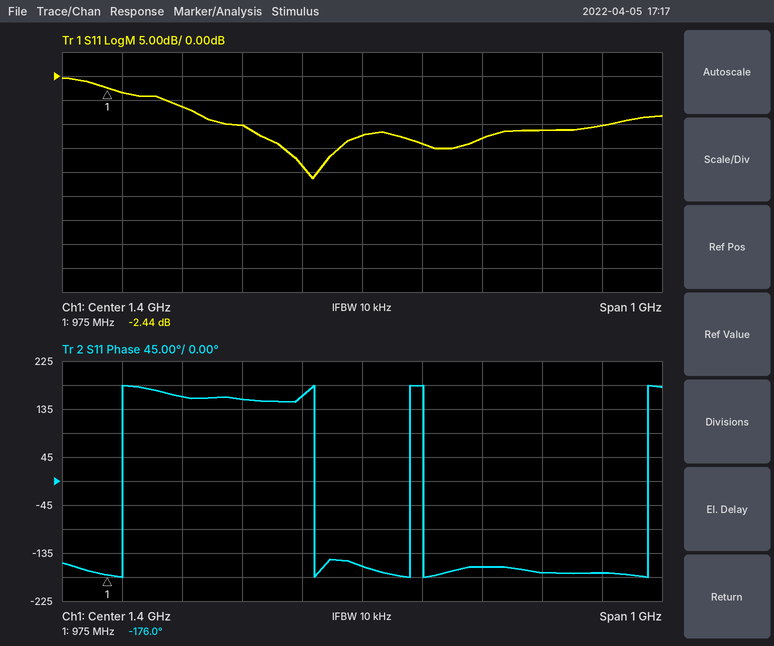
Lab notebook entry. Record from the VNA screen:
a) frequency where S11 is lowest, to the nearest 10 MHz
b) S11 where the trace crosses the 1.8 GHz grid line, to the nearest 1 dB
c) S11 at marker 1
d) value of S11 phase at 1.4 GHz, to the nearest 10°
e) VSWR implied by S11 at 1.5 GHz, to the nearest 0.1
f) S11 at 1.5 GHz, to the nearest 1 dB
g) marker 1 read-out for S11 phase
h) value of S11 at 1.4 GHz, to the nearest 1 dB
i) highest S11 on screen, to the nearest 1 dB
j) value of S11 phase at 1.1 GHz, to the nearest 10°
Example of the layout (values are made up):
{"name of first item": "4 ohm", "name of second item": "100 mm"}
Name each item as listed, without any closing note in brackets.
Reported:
{"frequency where S11 is lowest, to the nearest 10 MHz": "1.32 GHz", "S11 where the trace crosses the 1.8 GHz grid line, to the nearest 1 dB": "-10 dB", "S11 at marker 1": "-2.44 dB", "value of S11 phase at 1.4 GHz, to the nearest 10°": "-160°", "VSWR implied by S11 at 1.5 GHz, to the nearest 0.1": "1.5", "S11 at 1.5 GHz, to the nearest 1 dB": "-14 dB", "marker 1 read-out for S11 phase": "-176.0°", "value of S11 at 1.4 GHz, to the nearest 1 dB": "-12 dB", "highest S11 on screen, to the nearest 1 dB": "0 dB", "value of S11 phase at 1.1 GHz, to the nearest 10°": "160°"}
